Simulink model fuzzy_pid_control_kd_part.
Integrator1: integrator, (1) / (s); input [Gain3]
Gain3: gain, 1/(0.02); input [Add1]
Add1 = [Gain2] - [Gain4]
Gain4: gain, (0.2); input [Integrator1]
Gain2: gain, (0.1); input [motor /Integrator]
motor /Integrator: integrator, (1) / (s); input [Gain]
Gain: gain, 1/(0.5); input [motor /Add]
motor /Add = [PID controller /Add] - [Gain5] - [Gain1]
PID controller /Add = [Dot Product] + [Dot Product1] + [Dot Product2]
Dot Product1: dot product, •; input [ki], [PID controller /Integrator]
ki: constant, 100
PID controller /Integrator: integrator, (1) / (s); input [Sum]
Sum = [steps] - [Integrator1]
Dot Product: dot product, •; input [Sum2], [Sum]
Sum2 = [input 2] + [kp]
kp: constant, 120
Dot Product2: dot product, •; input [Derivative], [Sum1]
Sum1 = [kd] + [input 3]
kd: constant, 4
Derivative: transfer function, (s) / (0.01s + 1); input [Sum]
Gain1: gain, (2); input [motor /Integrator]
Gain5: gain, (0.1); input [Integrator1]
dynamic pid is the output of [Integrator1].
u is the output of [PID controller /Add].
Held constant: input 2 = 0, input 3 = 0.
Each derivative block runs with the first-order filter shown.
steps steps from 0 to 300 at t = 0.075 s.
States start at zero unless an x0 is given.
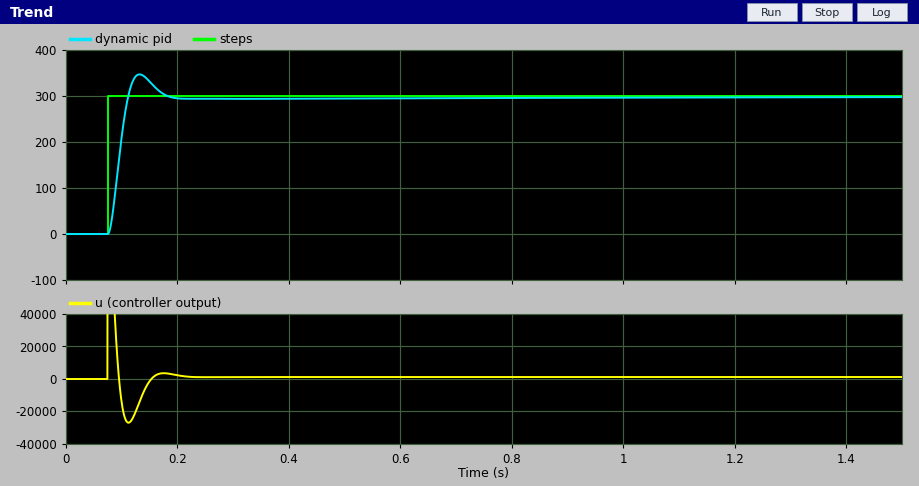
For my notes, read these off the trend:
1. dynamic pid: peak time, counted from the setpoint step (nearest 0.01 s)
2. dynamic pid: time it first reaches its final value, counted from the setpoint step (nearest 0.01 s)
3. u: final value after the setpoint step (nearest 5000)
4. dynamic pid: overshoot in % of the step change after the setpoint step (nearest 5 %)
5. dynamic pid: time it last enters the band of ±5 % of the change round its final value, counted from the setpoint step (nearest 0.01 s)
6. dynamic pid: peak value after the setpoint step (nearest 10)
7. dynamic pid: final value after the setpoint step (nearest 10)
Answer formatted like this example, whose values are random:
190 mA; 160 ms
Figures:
0.06 s; 0.04 s; 0; 15 %; 0.09 s; 350; 300
